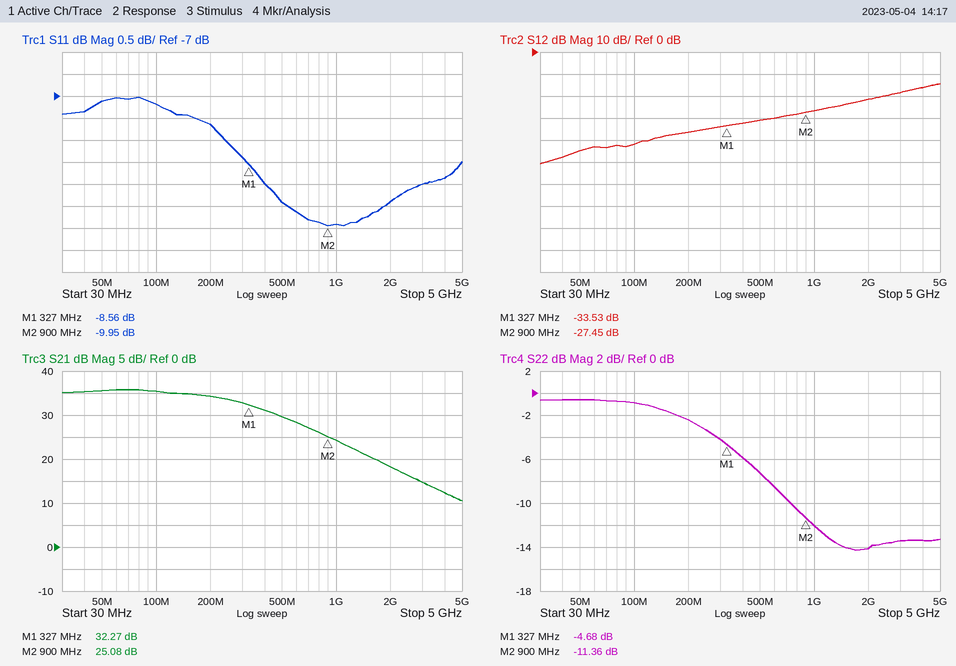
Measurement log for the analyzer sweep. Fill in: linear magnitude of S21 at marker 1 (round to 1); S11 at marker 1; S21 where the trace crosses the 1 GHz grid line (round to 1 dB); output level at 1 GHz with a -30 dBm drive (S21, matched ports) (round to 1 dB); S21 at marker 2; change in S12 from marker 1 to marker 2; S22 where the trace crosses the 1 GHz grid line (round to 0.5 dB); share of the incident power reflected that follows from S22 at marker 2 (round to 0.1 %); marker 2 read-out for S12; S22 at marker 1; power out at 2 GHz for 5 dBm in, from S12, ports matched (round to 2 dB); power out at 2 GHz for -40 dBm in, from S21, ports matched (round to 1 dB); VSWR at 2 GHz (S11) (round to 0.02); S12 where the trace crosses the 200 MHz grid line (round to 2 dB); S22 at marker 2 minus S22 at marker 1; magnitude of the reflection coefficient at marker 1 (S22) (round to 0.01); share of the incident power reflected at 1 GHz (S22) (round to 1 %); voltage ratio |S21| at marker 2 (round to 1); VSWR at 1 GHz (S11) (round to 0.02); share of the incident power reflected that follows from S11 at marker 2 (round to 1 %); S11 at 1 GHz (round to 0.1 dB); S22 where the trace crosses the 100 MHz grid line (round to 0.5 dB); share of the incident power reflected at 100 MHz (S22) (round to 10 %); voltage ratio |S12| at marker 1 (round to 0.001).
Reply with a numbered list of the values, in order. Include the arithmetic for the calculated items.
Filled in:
1. 10^(32.27/20) ≈ 41
2. -8.56 dB
3. 24 dB
4. -30 dBm + (24 dB) = -6 dBm
5. 25.08 dB
6. -27.45 − (-33.53) = 6.08 dB
7. -12.0 dB
8. 10^(-11.36/10) ≈ 7.3 %
9. -27.45 dB
10. -4.68 dB
11. 5 dBm + (-22 dB) = -16 dBm
12. -40 dBm + (18 dB) = -22 dBm
13. |Γ| = 10^(-9.4/20) = 0.3388; VSWR = (1 + 0.3388)/(1 − 0.3388) ≈ 2.03, so 2.02 to the nearest 0.02
14. -36 dB
15. -11.36 − (-4.68) = -6.68 dB
16. 10^(-4.68/20) ≈ 0.58
17. 10^(-12/10) ≈ 6 %
18. 10^(25.08/20) ≈ 18
19. |Γ| = 10^(-9.9/20) = 0.3199; VSWR = (1 + 0.3199)/(1 − 0.3199) ≈ 1.94
20. 10^(-9.95/10) ≈ 10 %
21. -9.9 dB
22. -1.0 dB
23. 10^(-1/10) ≈ 79.4 %, so 80 % to the nearest 10 %
24. 10^(-33.53/20) ≈ 0.021
